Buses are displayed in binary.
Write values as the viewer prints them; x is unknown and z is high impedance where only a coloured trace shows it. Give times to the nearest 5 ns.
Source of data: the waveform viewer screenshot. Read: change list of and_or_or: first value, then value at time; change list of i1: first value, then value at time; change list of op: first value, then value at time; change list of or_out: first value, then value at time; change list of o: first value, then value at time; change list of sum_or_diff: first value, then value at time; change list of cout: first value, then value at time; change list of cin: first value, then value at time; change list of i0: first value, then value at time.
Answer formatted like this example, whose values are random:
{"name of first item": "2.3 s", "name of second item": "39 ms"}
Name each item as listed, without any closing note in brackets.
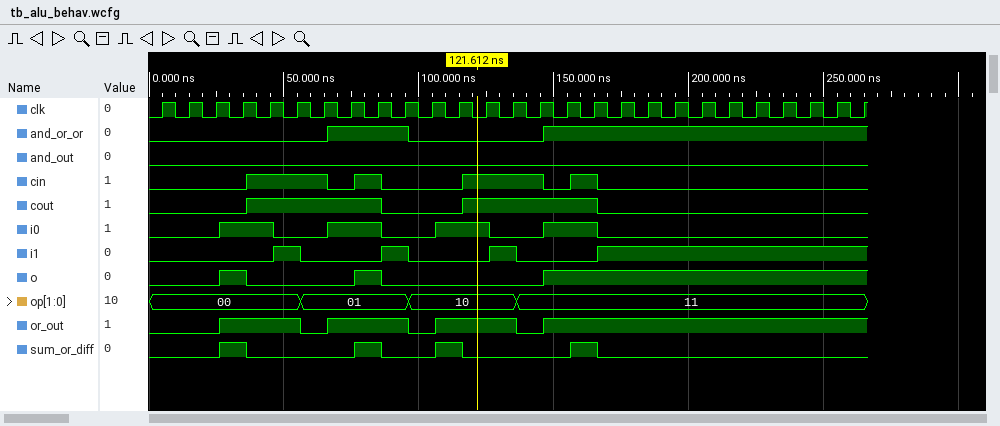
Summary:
{"change list of and_or_or: first value, then value at time": "0, 1 at 65 ns, 0 at 95 ns, 1 at 145 ns", "change list of i1: first value, then value at time": "0, 1 at 45 ns, 0 at 55 ns, 1 at 85 ns, 0 at 95 ns, 1 at 125 ns, 0 at 135 ns, 1 at 165 ns", "change list of op: first value, then value at time": "00, 01 at 55 ns, 10 at 95 ns, 11 at 135 ns", "change list of or_out: first value, then value at time": "0, 1 at 25 ns, 0 at 55 ns, 1 at 65 ns, 0 at 95 ns, 1 at 105 ns, 0 at 135 ns, 1 at 145 ns", "change list of o: first value, then value at time": "0, 1 at 25 ns, 0 at 35 ns, 1 at 75 ns, 0 at 85 ns, 1 at 145 ns", "change list of sum_or_diff: first value, then value at time": "0, 1 at 25 ns, 0 at 35 ns, 1 at 75 ns, 0 at 85 ns, 1 at 105 ns, 0 at 115 ns, 1 at 155 ns, 0 at 165 ns", "change list of cout: first value, then value at time": "0, 1 at 35 ns, 0 at 85 ns, 1 at 115 ns, 0 at 165 ns", "change list of cin: first value, then value at time": "0, 1 at 35 ns, 0 at 65 ns, 1 at 75 ns, 0 at 85 ns, 1 at 115 ns, 0 at 145 ns, 1 at 155 ns, 0 at 165 ns", "change list of i0: first value, then value at time": "0, 1 at 25 ns, 0 at 45 ns, 1 at 65 ns, 0 at 85 ns, 1 at 105 ns, 0 at 125 ns, 1 at 145 ns, 0 at 165 ns"}
